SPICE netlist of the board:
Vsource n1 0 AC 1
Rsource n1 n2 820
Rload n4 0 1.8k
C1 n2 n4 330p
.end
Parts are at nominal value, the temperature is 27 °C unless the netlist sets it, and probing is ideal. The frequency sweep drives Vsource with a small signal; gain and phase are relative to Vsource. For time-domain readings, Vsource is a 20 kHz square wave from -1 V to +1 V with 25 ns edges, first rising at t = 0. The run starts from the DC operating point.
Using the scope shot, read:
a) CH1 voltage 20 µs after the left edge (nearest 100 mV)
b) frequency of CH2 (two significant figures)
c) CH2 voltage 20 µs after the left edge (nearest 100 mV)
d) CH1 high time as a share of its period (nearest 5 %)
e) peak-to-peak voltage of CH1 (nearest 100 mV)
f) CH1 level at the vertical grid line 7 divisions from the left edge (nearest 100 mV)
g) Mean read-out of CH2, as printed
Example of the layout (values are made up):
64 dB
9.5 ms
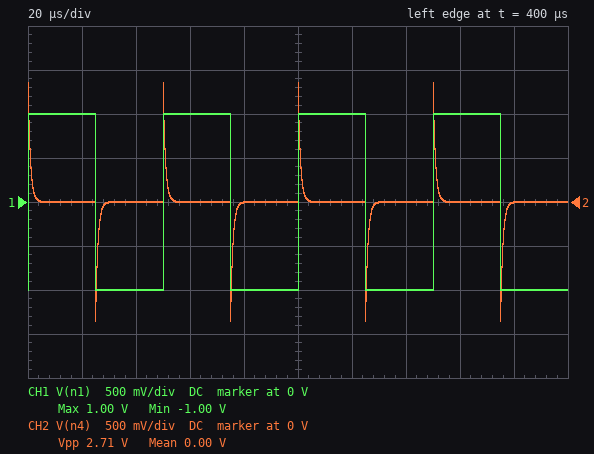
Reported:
1.0 V
20 kHz
0 V
50 %
2.0 V
-1.0 V
0.00 V
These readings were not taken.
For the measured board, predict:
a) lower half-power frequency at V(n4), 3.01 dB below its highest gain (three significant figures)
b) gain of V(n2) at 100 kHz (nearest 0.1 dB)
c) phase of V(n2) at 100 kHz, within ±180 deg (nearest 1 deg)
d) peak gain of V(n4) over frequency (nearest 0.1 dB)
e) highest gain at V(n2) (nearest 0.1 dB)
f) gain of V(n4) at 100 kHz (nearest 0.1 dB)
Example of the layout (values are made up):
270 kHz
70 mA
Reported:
184 kHz
-0.6 dB
-8 deg
-3.3 dB
0 dB
-9.7 dB
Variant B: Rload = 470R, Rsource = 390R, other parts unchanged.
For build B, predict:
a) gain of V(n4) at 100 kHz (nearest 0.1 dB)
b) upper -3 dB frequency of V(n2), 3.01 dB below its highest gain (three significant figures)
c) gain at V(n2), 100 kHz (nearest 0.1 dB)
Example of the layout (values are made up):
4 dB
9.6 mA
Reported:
-20.4 dB
884 kHz
-0.1 dB
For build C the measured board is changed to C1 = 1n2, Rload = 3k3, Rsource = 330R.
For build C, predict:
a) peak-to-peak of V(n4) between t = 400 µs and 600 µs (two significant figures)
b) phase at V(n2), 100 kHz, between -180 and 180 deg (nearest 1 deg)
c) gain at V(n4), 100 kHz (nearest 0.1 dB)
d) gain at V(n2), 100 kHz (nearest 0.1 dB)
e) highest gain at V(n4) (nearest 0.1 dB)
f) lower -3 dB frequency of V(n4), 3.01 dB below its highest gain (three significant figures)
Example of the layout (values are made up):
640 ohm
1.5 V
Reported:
3.6 V
-2 deg
-1.4 dB
-0.7 dB
-0.8 dB
36.5 kHz
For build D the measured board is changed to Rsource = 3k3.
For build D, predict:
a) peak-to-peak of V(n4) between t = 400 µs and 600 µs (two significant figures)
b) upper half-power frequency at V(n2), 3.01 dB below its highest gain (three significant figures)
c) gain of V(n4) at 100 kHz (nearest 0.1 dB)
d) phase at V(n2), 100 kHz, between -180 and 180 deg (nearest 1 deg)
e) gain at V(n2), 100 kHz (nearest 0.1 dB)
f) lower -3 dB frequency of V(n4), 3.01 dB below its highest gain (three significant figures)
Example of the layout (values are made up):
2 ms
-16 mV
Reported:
1.4 V
109 kHz
-11.8 dB
-26 deg
-2.7 dB
94.6 kHz
